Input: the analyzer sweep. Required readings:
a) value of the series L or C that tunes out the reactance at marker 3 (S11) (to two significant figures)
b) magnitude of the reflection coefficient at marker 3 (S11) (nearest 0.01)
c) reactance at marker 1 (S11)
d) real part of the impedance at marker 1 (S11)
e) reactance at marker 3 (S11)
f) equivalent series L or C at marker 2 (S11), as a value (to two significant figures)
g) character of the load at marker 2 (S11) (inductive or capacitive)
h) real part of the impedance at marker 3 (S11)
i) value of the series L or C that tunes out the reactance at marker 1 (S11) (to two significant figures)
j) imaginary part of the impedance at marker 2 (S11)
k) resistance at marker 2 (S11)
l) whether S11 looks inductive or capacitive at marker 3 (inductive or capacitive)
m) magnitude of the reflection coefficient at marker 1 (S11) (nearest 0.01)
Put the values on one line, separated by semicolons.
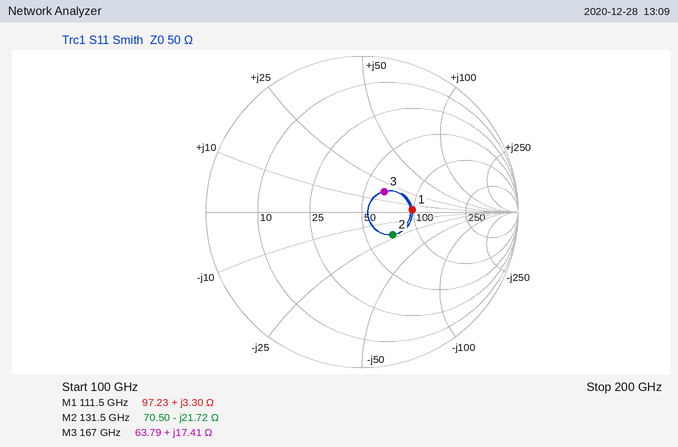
55 fF; 0.19; +3.30 Ω; 97.23 Ω; +17.41 Ω; 56 fF; capacitive; 63.79 Ω; 430 fF; -21.72 Ω; 70.50 Ω; inductive; 0.32
